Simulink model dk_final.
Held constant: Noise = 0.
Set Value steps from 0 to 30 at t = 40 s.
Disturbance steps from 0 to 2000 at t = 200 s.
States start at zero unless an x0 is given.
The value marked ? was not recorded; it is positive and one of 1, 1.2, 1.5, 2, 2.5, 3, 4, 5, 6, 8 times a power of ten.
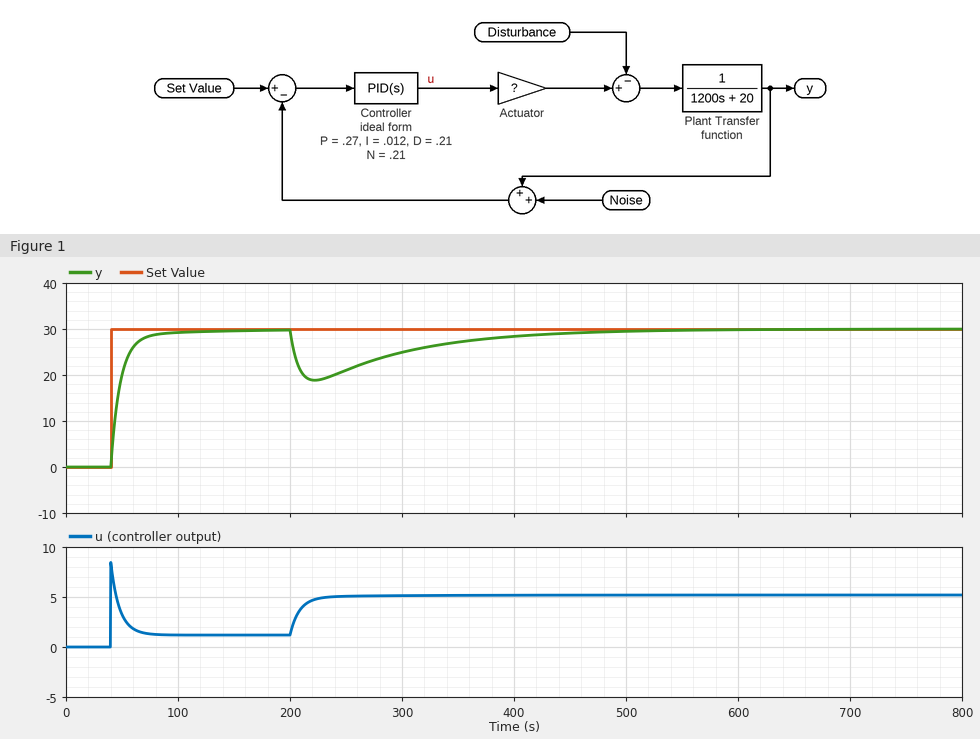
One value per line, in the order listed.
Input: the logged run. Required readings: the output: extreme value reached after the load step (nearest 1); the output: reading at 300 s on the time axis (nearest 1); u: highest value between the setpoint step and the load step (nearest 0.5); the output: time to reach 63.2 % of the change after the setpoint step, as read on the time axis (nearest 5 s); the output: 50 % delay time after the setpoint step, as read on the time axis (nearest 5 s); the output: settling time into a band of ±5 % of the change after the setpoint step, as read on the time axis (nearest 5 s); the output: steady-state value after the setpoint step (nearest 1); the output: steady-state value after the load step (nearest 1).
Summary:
19
25
8.5
50 s
45 s
75 s
30
30
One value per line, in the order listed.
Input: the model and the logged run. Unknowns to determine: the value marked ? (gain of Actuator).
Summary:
500
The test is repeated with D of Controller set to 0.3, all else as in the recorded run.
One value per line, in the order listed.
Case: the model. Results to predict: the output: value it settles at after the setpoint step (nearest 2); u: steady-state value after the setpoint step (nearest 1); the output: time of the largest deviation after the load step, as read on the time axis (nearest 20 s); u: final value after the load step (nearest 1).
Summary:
30
1
220 s
5
